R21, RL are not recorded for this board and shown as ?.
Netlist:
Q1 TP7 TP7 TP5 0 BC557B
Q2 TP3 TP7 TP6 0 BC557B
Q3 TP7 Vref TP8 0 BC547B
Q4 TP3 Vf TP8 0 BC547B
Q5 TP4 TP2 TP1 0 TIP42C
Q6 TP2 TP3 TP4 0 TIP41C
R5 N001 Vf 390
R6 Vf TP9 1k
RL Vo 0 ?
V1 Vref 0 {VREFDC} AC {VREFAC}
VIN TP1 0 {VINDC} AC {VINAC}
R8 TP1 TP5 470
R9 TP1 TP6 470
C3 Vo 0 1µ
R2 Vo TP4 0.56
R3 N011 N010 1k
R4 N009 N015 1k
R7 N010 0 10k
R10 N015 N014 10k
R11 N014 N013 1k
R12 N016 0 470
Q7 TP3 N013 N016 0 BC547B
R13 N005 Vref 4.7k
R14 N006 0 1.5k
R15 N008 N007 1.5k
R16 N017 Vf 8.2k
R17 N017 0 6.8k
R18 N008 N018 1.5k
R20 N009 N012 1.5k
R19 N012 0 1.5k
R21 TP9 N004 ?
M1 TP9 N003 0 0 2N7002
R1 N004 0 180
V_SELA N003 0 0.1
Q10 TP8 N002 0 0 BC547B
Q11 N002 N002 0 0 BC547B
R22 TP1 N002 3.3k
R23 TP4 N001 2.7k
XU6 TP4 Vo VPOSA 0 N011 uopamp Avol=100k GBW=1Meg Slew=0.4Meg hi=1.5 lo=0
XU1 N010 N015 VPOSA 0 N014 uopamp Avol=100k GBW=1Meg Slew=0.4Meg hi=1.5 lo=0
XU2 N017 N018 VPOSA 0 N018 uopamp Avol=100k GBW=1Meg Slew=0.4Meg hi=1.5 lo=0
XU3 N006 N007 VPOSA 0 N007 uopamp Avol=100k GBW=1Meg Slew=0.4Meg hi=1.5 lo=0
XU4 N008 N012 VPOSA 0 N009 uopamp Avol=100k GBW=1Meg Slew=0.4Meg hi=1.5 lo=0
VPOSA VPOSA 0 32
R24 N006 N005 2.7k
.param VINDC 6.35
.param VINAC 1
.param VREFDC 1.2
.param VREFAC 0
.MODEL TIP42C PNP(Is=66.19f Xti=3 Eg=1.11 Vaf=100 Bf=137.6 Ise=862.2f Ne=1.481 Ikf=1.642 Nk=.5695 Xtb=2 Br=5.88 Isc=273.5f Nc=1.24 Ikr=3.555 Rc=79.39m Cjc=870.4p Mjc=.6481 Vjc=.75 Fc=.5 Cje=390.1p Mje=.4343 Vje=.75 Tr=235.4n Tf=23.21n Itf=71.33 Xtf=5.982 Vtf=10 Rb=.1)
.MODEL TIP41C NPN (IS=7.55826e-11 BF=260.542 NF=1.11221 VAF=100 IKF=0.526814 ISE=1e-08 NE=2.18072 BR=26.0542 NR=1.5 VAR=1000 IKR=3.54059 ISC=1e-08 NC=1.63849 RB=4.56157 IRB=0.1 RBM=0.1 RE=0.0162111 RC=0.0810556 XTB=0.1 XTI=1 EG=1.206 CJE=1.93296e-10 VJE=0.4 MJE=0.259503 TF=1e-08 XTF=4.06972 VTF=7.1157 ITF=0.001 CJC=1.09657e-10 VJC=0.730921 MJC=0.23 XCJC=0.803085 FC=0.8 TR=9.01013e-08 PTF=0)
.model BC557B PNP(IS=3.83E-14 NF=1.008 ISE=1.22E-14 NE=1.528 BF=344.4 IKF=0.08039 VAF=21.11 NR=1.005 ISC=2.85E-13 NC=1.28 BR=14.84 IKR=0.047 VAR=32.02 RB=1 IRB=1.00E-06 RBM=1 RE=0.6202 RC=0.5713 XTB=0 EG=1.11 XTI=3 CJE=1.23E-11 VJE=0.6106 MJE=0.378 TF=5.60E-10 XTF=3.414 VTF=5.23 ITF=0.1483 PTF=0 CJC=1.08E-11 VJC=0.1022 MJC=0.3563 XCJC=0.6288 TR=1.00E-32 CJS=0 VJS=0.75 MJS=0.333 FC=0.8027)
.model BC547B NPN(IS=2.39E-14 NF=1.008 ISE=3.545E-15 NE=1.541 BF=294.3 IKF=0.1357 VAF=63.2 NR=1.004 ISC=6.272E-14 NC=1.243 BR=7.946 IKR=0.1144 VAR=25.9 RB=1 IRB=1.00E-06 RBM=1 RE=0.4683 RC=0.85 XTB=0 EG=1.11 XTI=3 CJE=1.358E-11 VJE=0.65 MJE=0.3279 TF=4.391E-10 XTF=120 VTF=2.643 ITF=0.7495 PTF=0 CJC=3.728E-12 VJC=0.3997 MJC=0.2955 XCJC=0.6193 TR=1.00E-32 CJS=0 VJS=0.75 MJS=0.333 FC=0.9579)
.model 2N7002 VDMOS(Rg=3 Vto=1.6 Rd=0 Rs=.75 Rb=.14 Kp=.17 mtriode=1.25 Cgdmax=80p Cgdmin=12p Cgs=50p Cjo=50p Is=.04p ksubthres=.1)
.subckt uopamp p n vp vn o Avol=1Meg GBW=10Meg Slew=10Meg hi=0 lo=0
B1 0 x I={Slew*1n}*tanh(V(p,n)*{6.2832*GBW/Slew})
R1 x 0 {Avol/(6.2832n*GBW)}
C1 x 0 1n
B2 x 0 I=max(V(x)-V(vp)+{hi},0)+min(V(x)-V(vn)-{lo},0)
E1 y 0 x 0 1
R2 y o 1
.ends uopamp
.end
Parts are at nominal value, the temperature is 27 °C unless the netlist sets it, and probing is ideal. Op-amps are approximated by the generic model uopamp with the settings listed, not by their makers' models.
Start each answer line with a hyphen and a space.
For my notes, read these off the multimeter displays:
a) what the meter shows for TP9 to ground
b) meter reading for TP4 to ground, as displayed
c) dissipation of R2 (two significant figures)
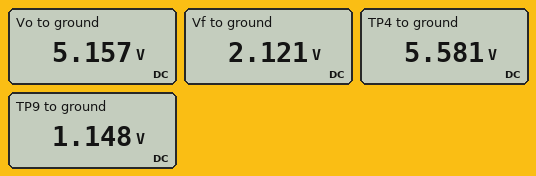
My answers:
- 1.148 V
- 5.581 V
- 320 mW
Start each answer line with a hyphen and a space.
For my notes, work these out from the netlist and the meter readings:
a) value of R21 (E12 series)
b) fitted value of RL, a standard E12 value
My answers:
- 1 kΩ
- 6.8 Ω
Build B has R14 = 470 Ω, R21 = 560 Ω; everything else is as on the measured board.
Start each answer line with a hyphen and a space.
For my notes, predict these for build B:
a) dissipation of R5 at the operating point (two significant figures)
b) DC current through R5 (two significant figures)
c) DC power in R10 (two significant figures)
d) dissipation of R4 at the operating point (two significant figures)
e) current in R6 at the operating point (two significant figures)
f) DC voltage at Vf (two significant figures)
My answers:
- 560 µW
- 1.2 mA
- 72 mW
- 7.2 mW
- 1.1 mA
- 1.9 V
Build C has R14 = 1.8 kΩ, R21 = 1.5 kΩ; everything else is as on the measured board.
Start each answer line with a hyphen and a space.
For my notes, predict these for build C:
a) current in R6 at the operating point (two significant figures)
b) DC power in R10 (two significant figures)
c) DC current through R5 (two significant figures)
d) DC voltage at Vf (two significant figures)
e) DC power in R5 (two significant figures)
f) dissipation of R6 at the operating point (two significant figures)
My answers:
- 880 µA
- 70 mW
- 1.0 mA
- 2.4 V
- 420 µW
- 770 µW
